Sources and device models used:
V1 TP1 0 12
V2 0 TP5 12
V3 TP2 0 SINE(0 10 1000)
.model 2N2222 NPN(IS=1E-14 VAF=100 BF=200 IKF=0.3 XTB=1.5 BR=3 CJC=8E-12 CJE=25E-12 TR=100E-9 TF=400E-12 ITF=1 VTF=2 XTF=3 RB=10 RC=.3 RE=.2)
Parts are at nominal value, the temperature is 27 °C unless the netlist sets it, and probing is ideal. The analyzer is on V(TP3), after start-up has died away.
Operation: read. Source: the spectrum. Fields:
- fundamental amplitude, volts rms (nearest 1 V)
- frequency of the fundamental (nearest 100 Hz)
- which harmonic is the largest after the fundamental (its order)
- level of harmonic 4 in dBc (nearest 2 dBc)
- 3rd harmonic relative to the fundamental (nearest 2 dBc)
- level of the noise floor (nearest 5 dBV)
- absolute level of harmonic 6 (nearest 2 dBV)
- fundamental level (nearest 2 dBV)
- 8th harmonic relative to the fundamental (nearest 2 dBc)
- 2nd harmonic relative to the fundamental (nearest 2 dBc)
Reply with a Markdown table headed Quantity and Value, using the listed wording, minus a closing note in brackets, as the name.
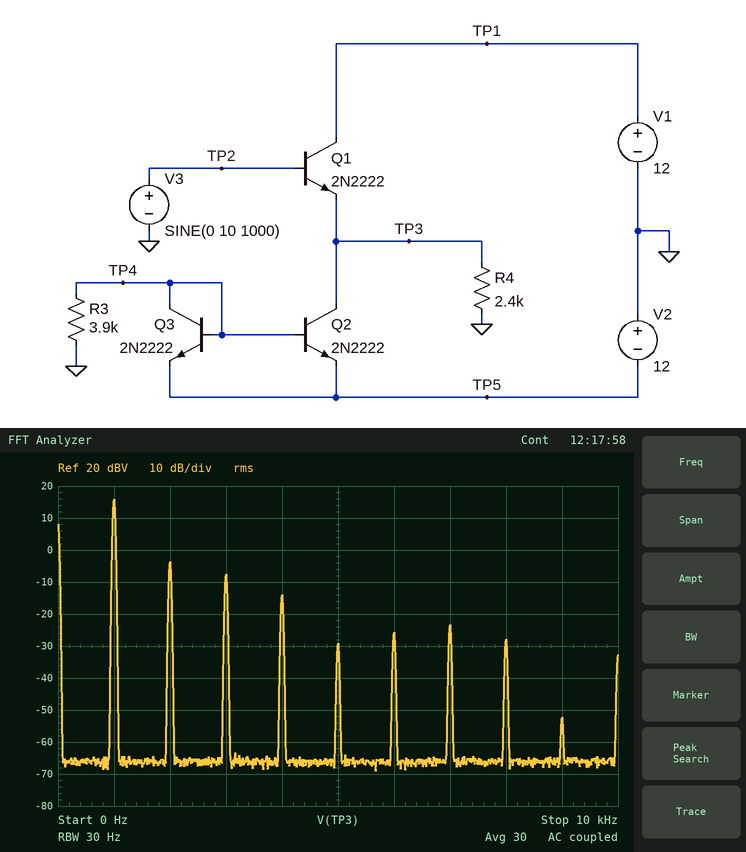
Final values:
| Quantity | Value |
|---|---|
| fundamental amplitude, volts rms | 6 V |
| frequency of the fundamental | 1.0 kHz |
| which harmonic is the largest after the fundamental | 2 |
| level of harmonic 4 in dBc | -30 dBc |
| 3rd harmonic relative to the fundamental | -24 dBc |
| level of the noise floor | -65 dBV |
| absolute level of harmonic 6 | -26 dBV |
| fundamental level | 16 dBV |
| 8th harmonic relative to the fundamental | -44 dBc |
| 2nd harmonic relative to the fundamental | -20 dBc |
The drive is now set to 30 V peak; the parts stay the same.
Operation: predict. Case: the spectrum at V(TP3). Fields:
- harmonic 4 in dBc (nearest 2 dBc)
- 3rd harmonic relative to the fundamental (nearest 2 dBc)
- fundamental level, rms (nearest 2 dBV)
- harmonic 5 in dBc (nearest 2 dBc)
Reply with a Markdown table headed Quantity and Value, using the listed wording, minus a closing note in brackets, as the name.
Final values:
| Quantity | Value |
|---|---|
| harmonic 4 in dBc | -22 dBc |
| 3rd harmonic relative to the fundamental | -12 dBc |
| fundamental level, rms | 18 dBV |
| harmonic 5 in dBc | -20 dBc |
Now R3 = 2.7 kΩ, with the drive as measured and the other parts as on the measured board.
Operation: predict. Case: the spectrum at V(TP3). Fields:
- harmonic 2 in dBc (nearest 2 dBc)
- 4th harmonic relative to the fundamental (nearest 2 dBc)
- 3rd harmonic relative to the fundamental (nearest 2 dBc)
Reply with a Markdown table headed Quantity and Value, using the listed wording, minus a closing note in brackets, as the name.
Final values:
| Quantity | Value |
|---|---|
| harmonic 2 in dBc | -40 dBc |
| 4th harmonic relative to the fundamental | -44 dBc |
| 3rd harmonic relative to the fundamental | -42 dBc |
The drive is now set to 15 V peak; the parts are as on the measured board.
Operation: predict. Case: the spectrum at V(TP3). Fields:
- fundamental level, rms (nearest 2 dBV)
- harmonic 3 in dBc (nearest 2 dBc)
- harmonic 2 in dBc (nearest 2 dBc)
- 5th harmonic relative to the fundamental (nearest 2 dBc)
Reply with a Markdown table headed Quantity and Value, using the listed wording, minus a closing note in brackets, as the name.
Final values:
| Quantity | Value |
|---|---|
| fundamental level, rms | 18 dBV |
| harmonic 3 in dBc | -18 dBc |
| harmonic 2 in dBc | -16 dBc |
| 5th harmonic relative to the fundamental | -42 dBc |
